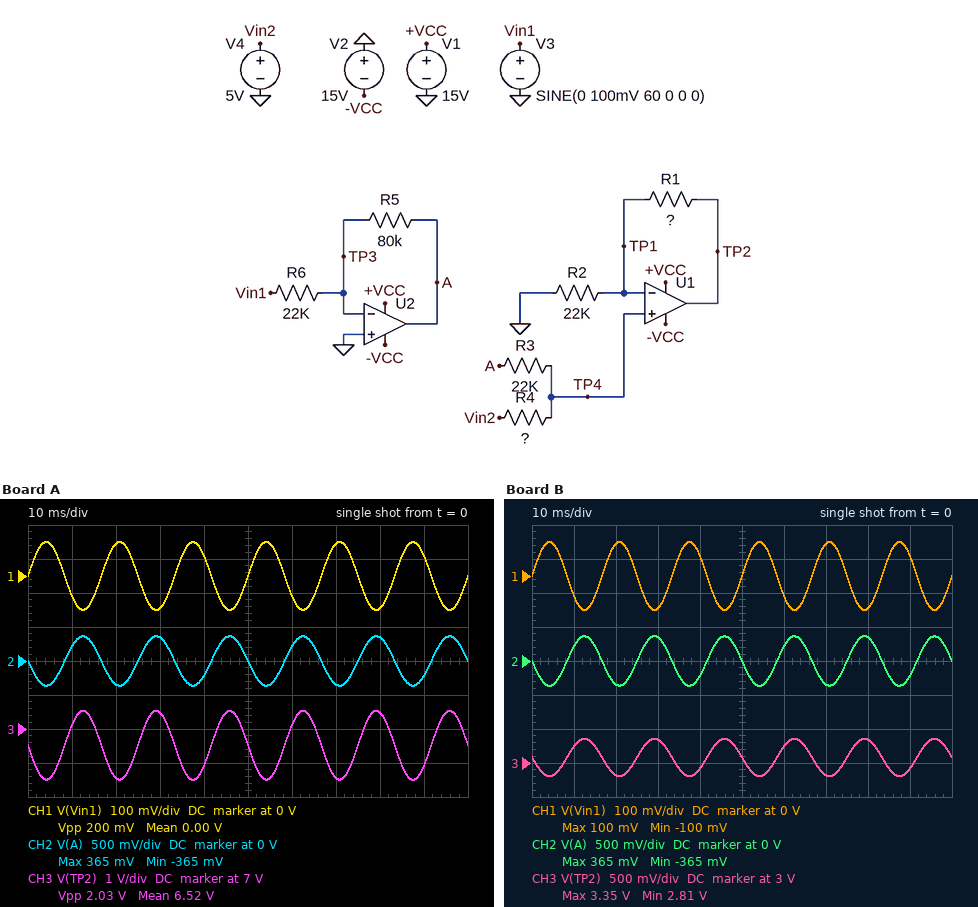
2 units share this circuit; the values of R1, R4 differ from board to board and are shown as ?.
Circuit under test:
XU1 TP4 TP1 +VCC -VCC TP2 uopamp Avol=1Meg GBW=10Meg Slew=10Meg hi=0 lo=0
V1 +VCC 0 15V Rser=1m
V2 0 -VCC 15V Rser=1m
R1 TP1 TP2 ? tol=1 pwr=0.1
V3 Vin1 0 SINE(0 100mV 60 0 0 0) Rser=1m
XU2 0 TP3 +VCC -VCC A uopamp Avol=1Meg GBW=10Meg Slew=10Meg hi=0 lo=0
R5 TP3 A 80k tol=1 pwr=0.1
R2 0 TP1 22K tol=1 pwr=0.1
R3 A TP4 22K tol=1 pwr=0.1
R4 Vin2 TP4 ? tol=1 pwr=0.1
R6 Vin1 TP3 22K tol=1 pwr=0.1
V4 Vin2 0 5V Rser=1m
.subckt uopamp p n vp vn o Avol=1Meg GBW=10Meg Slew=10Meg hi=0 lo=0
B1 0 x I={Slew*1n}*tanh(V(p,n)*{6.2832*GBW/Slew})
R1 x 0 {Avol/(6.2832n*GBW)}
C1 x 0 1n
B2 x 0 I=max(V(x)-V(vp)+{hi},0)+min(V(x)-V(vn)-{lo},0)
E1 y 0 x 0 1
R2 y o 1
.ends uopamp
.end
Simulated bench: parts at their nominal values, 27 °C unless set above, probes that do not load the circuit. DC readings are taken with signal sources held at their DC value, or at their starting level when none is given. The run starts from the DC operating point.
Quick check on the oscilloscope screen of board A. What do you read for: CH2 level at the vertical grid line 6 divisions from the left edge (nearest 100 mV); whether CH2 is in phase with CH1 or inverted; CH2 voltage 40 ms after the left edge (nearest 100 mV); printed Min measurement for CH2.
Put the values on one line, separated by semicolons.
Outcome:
200 mV; inverted; -200 mV; -365 mV
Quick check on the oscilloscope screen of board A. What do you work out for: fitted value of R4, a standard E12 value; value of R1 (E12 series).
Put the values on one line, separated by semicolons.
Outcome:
47 kΩ; 68 kΩ
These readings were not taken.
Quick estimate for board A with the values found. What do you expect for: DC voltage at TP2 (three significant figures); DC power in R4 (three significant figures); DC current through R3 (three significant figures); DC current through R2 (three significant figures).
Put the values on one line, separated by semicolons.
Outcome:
6.52 V; 247 µW; 72.5 µA; 72.5 µA
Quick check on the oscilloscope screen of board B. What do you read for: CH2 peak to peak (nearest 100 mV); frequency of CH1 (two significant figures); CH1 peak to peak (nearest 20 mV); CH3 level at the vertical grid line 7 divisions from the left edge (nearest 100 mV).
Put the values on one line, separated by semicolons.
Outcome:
700 mV; 60 Hz; 200 mV; 2.8 V
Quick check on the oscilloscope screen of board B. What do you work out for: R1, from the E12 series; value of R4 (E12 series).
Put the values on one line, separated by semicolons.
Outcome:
8.2 kΩ; 27 kΩ
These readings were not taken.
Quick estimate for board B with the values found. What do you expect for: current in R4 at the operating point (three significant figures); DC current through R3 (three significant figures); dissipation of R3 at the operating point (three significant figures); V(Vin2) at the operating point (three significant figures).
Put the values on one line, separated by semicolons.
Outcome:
102 µA; 102 µA; 229 µW; 5.00 V
